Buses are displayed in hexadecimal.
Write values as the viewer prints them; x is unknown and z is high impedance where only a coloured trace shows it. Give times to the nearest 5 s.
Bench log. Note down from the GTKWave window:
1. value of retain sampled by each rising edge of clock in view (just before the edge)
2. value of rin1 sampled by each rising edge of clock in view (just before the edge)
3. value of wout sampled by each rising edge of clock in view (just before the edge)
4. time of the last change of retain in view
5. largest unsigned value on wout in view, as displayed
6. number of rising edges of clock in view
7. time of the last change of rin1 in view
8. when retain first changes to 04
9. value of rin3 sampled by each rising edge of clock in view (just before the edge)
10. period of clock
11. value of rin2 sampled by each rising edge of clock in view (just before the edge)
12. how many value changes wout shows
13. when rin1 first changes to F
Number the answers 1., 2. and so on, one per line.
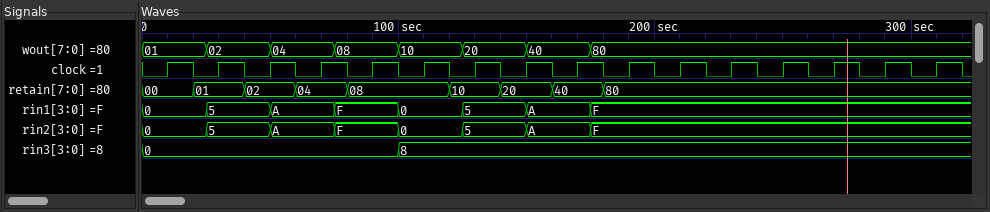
1. 00, 01, 02, 04, 08, 08, 10, 20, 40, 80, 80, 80, 80, 80, 80, 80
2. 0, 5, 5, A, F, 0, 5, 5, A, F, F, F, F, F, F, F
3. 01, 02, 02, 04, 08, 10, 20, 20, 40, 80, 80, 80, 80, 80, 80, 80
4. 180 s
5. 80
6. 16
7. 175 s
8. 60 s
9. 0, 0, 0, 0, 0, 8, 8, 8, 8, 8, 8, 8, 8, 8, 8, 8
10. 20 s
11. 0, 5, 5, A, F, 0, 5, 5, A, F, F, F, F, F, F, F
12. 7
13. 75 s
